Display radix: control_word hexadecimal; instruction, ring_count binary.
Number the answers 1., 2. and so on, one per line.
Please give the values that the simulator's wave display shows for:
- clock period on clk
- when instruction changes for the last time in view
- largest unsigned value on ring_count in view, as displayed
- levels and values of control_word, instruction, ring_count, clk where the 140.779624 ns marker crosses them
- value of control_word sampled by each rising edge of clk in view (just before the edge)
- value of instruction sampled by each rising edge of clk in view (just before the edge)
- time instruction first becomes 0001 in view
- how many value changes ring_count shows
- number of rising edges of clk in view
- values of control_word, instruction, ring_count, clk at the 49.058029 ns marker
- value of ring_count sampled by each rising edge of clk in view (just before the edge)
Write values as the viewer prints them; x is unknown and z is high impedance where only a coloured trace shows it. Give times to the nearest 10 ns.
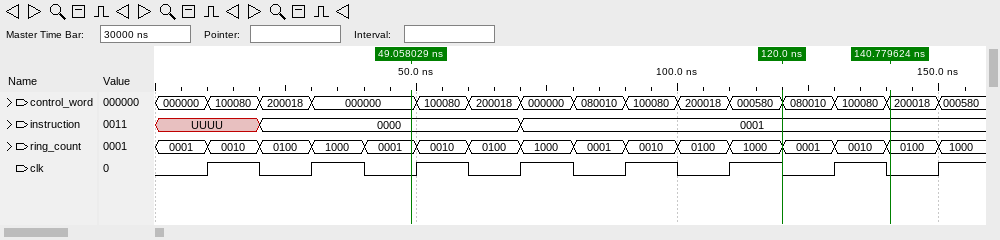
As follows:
1. 20 ns
2. 70 ns
3. 1000
4. control_word=200018, instruction=0001, ring_count=0100, clk=0
5. 000000, 200018, 000000, 200018, 080010, 200018, 080010, 200018
6. UUUU, 0000, 0000, 0000, 0001, 0001, 0001, 0001
7. 70 ns
8. 15
9. 8
10. control_word=000000, instruction=0000, ring_count=0001, clk=0
11. 0001, 0100, 0001, 0100, 0001, 0100, 0001, 0100
